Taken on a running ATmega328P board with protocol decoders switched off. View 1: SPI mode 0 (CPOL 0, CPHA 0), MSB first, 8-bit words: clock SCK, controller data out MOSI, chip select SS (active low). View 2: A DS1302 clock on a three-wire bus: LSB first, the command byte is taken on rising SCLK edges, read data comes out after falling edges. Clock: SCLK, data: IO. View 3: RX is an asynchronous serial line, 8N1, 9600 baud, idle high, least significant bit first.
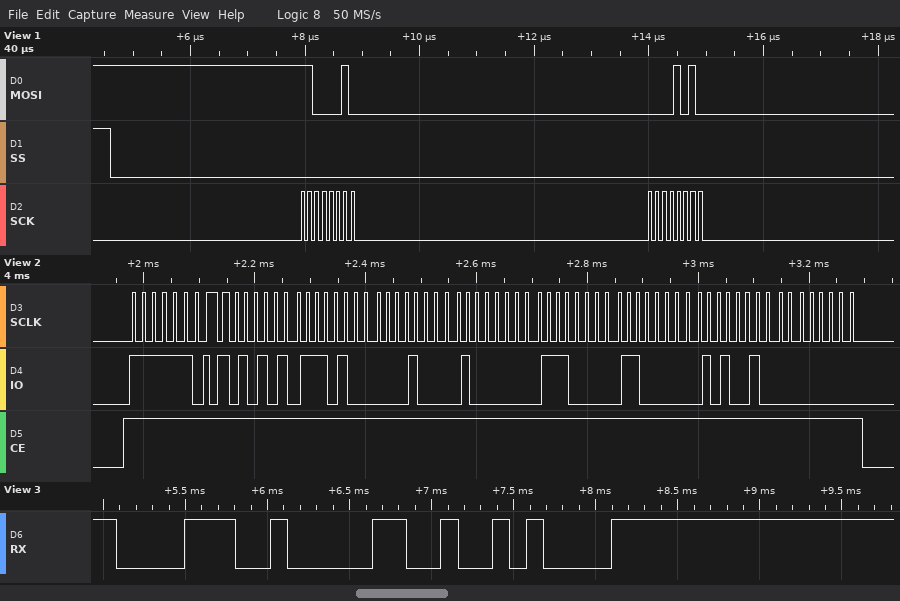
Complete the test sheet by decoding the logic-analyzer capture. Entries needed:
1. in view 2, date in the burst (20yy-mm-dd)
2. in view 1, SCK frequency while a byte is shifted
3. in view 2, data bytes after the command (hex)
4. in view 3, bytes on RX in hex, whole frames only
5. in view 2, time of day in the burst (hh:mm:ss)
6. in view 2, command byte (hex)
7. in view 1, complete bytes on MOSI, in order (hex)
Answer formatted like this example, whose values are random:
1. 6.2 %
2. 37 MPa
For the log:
1. 2025-07-01
2. 8 MHz
3. 55 17 08 01 07 03 25 00
4. 0x38 0x30 0x0A
5. 08:17:55
6. 0xBF
7. C2 0A
